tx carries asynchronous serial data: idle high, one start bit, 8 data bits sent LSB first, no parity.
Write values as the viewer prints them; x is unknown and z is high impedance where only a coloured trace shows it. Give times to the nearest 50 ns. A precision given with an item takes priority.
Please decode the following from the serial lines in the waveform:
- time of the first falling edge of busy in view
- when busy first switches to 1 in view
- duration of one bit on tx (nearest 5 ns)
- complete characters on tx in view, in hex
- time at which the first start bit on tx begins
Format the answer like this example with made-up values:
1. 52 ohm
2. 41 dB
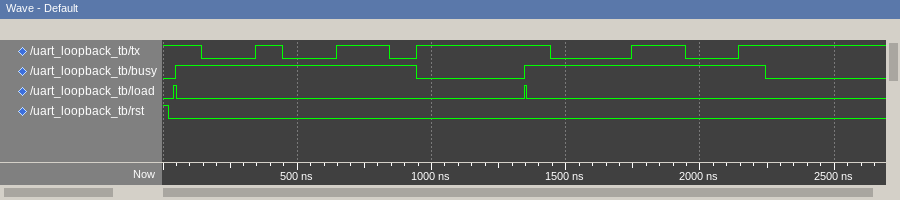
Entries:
1. 950 ns
2. 50 ns
3. 100 ns
4. B2, CC
5. 150 ns
